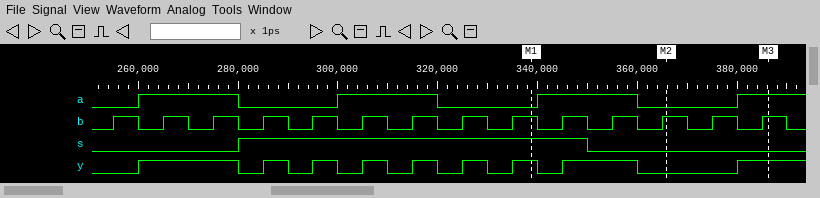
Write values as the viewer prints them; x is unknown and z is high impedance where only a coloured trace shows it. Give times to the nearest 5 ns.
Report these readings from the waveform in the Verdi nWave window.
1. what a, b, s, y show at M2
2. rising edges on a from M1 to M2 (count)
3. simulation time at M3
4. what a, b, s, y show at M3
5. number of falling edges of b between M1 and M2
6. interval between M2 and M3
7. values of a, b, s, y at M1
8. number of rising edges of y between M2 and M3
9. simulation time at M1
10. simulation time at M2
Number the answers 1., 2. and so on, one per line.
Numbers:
1. a=0, b=1, s=0, y=0
2. 1
3. 385 ns
4. a=1, b=1, s=0, y=1
5. 3
6. 20 ns
7. a=0, b=1, s=1, y=1
8. 1
9. 340 ns
10. 365 ns
